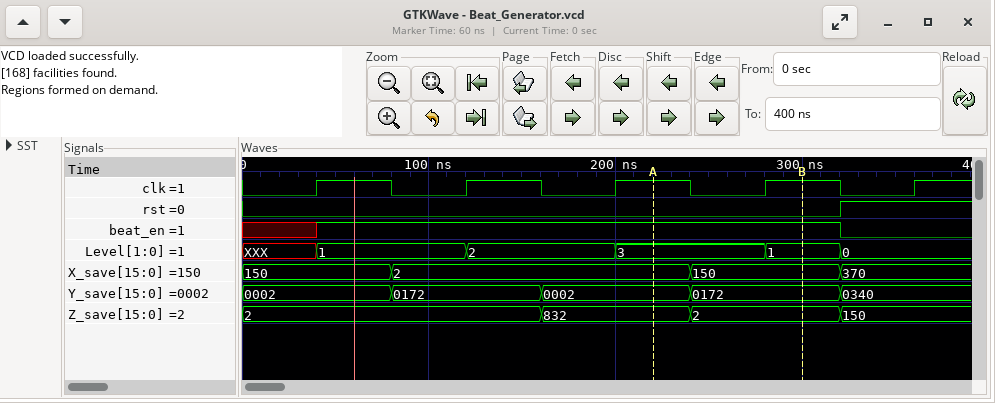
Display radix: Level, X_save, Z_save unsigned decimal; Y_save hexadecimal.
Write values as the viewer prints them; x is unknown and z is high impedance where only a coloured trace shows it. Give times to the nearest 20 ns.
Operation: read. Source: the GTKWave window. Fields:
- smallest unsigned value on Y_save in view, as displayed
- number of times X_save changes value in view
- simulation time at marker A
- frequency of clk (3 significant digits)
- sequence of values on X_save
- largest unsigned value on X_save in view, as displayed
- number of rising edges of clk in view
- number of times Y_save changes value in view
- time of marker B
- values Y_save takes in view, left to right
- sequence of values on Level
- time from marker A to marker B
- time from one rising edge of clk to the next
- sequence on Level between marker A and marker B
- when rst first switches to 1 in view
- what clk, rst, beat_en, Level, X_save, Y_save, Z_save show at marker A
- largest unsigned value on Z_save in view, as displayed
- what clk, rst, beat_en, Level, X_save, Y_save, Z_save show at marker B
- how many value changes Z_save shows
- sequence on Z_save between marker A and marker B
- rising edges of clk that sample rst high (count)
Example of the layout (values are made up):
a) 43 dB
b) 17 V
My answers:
a) 0002
b) 3
c) 220 ns
d) 12.5 MHz
e) 150, 2, 150, 370
f) 370
g) 5
h) 4
i) 300 ns
j) 0002, 0172, 0002, 0172, 0340
k) XXX, 1, 2, 3, 1, 0
l) 80 ns
m) 80 ns
n) 3, 1
o) 320 ns
p) clk=1, rst=0, beat_en=1, Level=3, X_save=2, Y_save=0002, Z_save=832
q) 832
r) clk=1, rst=0, beat_en=1, Level=1, X_save=150, Y_save=0172, Z_save=2
s) 3
t) 832, 2
u) 1
